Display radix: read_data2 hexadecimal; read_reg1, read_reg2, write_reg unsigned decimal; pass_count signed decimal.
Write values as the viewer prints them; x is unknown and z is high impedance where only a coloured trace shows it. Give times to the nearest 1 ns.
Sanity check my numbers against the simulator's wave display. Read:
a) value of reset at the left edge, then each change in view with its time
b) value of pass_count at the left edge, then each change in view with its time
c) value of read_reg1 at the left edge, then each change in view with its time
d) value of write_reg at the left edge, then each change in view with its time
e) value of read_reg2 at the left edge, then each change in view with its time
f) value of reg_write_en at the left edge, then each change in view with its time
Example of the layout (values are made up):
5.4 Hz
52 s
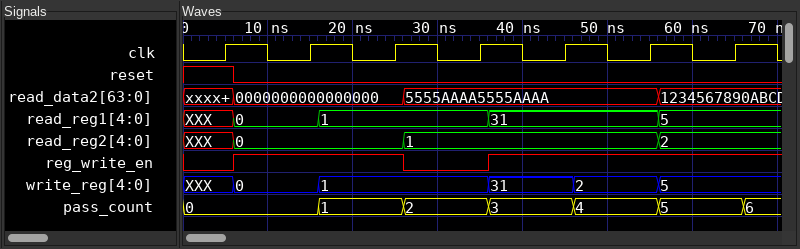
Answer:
1, 0 at 6 ns
0, 1 at 16 ns, 2 at 26 ns, 3 at 36 ns, 4 at 46 ns, 5 at 56 ns, 6 at 66 ns
XXX, 0 at 6 ns, 1 at 16 ns, 31 at 36 ns, 5 at 56 ns
XXX, 0 at 6 ns, 1 at 16 ns, 31 at 36 ns, 2 at 46 ns, 5 at 56 ns
XXX, 0 at 6 ns, 1 at 26 ns, 2 at 56 ns
0, 1 at 6 ns, 0 at 26 ns, 1 at 36 ns
